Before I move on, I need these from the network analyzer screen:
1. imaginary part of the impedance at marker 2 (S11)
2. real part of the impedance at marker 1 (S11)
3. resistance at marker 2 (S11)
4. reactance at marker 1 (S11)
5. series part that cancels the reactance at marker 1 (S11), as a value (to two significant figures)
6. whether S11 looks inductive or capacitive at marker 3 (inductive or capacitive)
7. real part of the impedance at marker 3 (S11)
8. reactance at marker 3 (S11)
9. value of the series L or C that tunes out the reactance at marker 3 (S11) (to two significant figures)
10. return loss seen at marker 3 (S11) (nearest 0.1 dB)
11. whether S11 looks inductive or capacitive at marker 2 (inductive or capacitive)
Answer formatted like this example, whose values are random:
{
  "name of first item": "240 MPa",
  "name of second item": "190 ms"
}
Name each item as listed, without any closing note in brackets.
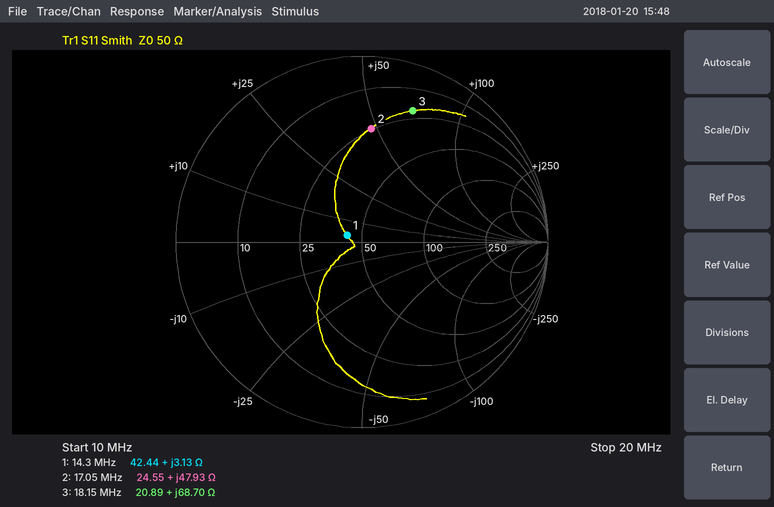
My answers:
{
  "imaginary part of the impedance at marker 2": "+47.93 Ω",
  "real part of the impedance at marker 1": "42.44 Ω",
  "resistance at marker 2": "24.55 Ω",
  "reactance at marker 1": "+3.13 Ω",
  "series part that cancels the reactance at marker 1 (S11), as a value": "3.6 nF",
  "whether S11 looks inductive or capacitive at marker 3": "inductive",
  "real part of the impedance at marker 3": "20.89 Ω",
  "reactance at marker 3": "+68.70 Ω",
  "value of the series L or C that tunes out the reactance at marker 3 (S11)": "130 pF",
  "return loss seen at marker 3 (S11)": "2.4 dB",
  "whether S11 looks inductive or capacitive at marker 2": "inductive"
}
